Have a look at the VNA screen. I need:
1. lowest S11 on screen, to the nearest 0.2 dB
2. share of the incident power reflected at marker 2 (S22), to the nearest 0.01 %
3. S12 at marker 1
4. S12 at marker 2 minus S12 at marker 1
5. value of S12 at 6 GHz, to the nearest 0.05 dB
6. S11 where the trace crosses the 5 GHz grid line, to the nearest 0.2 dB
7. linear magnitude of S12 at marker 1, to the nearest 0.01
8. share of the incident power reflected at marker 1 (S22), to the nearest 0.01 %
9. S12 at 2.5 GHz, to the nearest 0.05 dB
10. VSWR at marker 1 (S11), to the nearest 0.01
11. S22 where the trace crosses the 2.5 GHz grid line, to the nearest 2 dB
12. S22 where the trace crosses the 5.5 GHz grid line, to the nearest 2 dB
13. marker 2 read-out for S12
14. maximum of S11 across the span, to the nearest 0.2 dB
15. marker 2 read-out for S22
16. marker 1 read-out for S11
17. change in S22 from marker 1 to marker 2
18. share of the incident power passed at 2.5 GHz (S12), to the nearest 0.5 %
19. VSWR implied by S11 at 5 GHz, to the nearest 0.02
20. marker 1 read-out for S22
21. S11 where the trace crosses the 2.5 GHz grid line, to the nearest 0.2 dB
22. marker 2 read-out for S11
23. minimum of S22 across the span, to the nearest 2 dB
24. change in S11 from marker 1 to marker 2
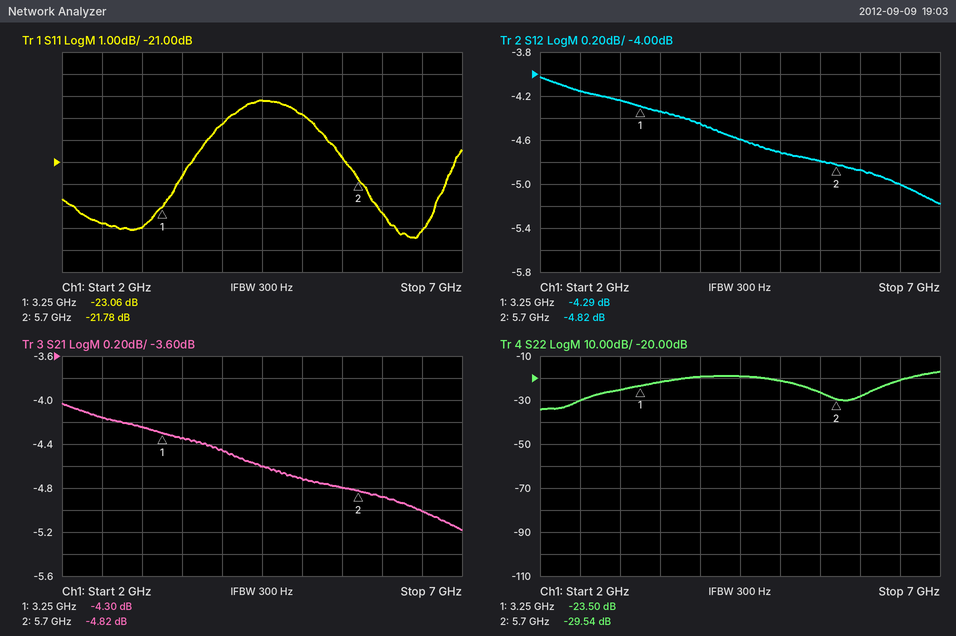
-24.4 dB
0.11 %
-4.29 dB
-0.53 dB
-4.85 dB
-18.8 dB
0.61
0.45 %
-4.15 dB
1.15
-30 dB
-26 dB
-4.82 dB
-18.2 dB
-29.54 dB
-23.06 dB
-6.04 dB
38.5 %
1.26
-23.50 dB
-23.8 dB
-21.78 dB
-34 dB
1.28 dB
